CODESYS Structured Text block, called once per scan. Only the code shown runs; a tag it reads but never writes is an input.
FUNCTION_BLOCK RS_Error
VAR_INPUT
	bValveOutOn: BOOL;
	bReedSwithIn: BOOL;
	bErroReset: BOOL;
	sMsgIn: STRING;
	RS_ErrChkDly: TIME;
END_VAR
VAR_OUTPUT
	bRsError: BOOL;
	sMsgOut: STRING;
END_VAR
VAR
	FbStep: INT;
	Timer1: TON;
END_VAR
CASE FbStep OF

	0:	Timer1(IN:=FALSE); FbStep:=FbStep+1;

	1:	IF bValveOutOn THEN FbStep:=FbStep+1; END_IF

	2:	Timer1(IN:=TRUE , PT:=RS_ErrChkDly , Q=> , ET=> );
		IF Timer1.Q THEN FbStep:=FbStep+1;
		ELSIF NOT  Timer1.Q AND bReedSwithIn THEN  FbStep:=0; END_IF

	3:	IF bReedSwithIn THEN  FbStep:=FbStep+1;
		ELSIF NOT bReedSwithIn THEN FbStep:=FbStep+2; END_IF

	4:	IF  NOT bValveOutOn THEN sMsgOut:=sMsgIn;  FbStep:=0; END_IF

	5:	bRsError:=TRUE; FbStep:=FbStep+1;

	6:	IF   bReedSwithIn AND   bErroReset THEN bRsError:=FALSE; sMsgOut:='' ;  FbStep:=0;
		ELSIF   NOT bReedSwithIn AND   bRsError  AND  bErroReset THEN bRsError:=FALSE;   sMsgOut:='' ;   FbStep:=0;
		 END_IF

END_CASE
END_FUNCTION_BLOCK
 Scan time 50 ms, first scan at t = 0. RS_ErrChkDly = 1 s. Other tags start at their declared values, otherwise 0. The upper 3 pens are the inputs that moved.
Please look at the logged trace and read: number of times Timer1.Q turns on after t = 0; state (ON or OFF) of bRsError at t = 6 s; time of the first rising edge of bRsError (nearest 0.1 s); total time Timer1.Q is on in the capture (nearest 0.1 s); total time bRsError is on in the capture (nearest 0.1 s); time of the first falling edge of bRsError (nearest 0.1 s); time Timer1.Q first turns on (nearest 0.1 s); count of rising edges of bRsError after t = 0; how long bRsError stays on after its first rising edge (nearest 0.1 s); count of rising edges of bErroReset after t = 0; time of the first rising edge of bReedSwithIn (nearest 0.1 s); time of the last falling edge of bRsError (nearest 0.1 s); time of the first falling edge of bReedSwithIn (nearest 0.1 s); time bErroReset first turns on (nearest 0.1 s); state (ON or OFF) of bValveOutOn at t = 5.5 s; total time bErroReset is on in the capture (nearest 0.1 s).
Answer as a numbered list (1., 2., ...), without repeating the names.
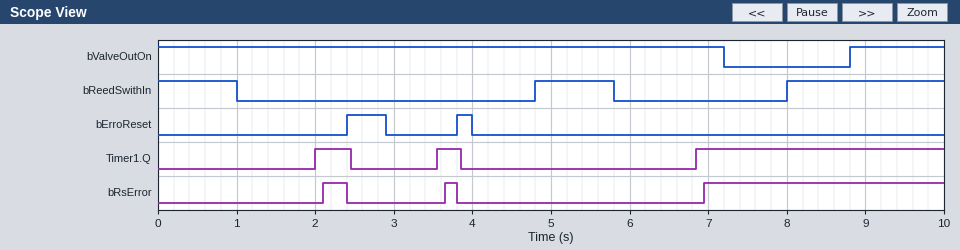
1. 3
2. OFF
3. 2.1 s
4. 3.9 s
5. 3.5 s
6. 2.4 s
7. 2.0 s
8. 3
9. 0.3 s
10. 2
11. 4.8 s
12. 3.8 s
13. 1.0 s
14. 2.4 s
15. ON
16. 0.7 s
